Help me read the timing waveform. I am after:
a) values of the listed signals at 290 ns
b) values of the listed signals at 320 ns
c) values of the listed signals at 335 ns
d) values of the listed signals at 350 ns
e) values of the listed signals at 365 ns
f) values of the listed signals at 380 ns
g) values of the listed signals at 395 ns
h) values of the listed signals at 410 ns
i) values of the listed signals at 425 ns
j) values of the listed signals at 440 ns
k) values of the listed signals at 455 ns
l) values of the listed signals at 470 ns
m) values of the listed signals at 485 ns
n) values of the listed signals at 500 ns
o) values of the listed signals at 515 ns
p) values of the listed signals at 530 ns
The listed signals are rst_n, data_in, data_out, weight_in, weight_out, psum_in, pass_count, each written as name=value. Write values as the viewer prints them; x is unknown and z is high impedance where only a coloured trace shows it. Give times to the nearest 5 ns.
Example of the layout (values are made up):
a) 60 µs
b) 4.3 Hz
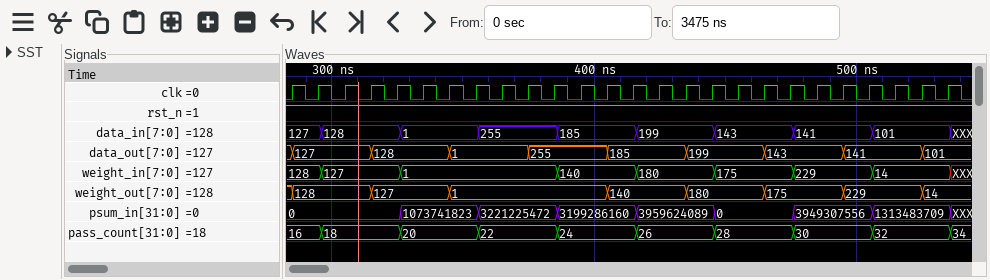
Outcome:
a) rst_n=1, data_in=127, data_out=127, weight_in=128, weight_out=128, psum_in=0, pass_count=16
b) rst_n=1, data_in=128, data_out=128, weight_in=127, weight_out=127, psum_in=0, pass_count=18
c) rst_n=1, data_in=1, data_out=128, weight_in=1, weight_out=127, psum_in=1073741823, pass_count=20
d) rst_n=1, data_in=1, data_out=1, weight_in=1, weight_out=1, psum_in=1073741823, pass_count=20
e) rst_n=1, data_in=255, data_out=1, weight_in=1, weight_out=1, psum_in=3221225472, pass_count=22
f) rst_n=1, data_in=255, data_out=255, weight_in=1, weight_out=1, psum_in=3221225472, pass_count=22
g) rst_n=1, data_in=185, data_out=255, weight_in=140, weight_out=1, psum_in=3199286160, pass_count=24
h) rst_n=1, data_in=185, data_out=185, weight_in=140, weight_out=140, psum_in=3199286160, pass_count=24
i) rst_n=1, data_in=199, data_out=185, weight_in=180, weight_out=140, psum_in=3959624089, pass_count=26
j) rst_n=1, data_in=199, data_out=199, weight_in=180, weight_out=180, psum_in=3959624089, pass_count=26
k) rst_n=1, data_in=143, data_out=199, weight_in=175, weight_out=180, psum_in=0, pass_count=28
l) rst_n=1, data_in=143, data_out=143, weight_in=175, weight_out=175, psum_in=0, pass_count=28
m) rst_n=1, data_in=141, data_out=143, weight_in=229, weight_out=175, psum_in=3949307556, pass_count=30
n) rst_n=1, data_in=141, data_out=141, weight_in=229, weight_out=229, psum_in=3949307556, pass_count=30
o) rst_n=1, data_in=101, data_out=141, weight_in=14, weight_out=229, psum_in=1313483709, pass_count=32
p) rst_n=1, data_in=101, data_out=101, weight_in=14, weight_out=14, psum_in=1313483709, pass_count=32
